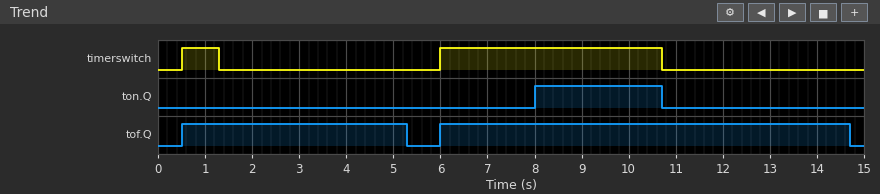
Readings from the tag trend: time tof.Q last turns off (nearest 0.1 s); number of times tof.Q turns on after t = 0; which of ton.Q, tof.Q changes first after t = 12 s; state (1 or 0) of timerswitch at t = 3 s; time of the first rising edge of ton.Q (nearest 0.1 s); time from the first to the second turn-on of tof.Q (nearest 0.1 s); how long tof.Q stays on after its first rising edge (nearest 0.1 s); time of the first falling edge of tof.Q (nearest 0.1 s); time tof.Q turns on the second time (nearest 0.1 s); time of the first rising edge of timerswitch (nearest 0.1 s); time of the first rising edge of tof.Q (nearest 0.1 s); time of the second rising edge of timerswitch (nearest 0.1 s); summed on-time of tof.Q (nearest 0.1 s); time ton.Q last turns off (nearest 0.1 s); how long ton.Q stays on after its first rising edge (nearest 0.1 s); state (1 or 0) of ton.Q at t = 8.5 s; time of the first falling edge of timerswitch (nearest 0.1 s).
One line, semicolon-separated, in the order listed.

14.7 s; 2; tof.Q; 0; 8.0 s; 5.5 s; 4.8 s; 5.3 s; 6.0 s; 0.5 s; 0.5 s; 6.0 s; 13.5 s; 10.7 s; 2.7 s; 1; 1.3 s
